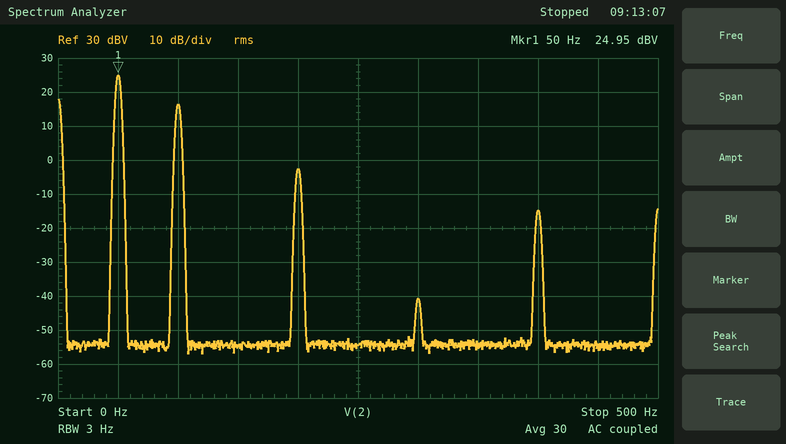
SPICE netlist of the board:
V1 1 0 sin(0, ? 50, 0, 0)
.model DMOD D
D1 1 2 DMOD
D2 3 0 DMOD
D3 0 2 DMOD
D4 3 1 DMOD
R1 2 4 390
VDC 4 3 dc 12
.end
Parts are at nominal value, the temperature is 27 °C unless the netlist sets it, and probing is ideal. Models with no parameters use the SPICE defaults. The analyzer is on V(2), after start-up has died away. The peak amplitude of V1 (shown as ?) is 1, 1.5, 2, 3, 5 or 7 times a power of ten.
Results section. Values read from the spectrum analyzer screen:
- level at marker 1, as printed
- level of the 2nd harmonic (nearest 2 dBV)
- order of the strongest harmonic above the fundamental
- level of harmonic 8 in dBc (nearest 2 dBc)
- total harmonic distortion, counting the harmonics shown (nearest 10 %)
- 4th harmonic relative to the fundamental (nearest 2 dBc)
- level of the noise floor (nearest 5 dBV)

24.95 dBV
16 dBV
2
-40 dBc
40 %
-28 dBc
-55 dBV
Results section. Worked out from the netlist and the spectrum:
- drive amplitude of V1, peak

50 V
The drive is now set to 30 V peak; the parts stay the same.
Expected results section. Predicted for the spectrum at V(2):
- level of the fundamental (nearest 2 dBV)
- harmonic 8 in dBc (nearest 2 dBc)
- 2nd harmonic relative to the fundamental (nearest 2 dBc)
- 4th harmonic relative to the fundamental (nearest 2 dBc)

20 dBV
-36 dBc
-10 dBc
-38 dBc
